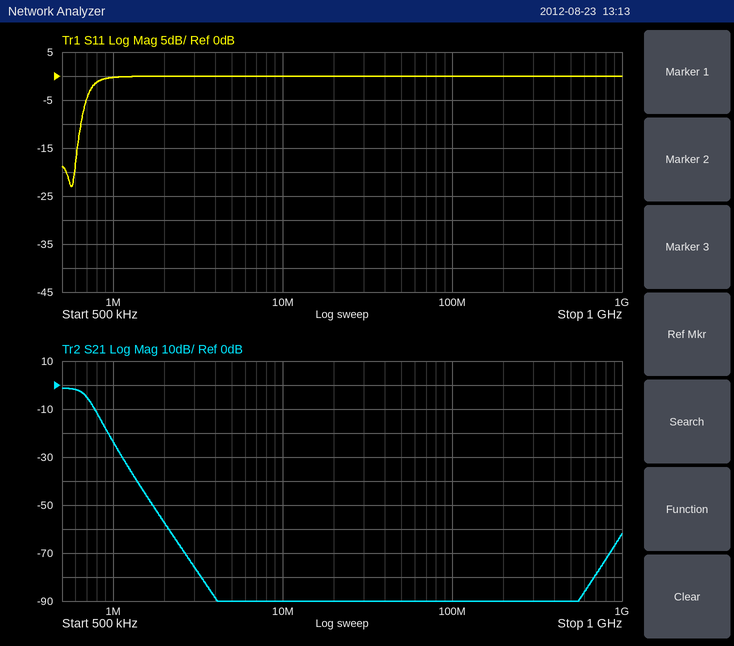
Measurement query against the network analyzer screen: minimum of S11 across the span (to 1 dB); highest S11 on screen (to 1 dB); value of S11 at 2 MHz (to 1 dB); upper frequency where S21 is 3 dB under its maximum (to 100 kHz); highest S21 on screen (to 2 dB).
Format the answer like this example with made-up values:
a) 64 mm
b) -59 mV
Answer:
a) -23 dB
b) 0 dB
c) 0 dB
d) 700 kHz
e) -2 dB
